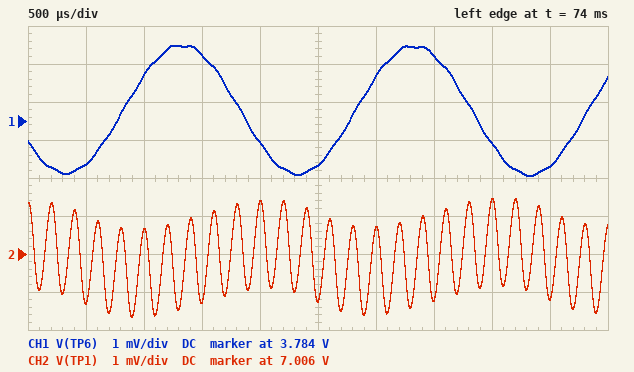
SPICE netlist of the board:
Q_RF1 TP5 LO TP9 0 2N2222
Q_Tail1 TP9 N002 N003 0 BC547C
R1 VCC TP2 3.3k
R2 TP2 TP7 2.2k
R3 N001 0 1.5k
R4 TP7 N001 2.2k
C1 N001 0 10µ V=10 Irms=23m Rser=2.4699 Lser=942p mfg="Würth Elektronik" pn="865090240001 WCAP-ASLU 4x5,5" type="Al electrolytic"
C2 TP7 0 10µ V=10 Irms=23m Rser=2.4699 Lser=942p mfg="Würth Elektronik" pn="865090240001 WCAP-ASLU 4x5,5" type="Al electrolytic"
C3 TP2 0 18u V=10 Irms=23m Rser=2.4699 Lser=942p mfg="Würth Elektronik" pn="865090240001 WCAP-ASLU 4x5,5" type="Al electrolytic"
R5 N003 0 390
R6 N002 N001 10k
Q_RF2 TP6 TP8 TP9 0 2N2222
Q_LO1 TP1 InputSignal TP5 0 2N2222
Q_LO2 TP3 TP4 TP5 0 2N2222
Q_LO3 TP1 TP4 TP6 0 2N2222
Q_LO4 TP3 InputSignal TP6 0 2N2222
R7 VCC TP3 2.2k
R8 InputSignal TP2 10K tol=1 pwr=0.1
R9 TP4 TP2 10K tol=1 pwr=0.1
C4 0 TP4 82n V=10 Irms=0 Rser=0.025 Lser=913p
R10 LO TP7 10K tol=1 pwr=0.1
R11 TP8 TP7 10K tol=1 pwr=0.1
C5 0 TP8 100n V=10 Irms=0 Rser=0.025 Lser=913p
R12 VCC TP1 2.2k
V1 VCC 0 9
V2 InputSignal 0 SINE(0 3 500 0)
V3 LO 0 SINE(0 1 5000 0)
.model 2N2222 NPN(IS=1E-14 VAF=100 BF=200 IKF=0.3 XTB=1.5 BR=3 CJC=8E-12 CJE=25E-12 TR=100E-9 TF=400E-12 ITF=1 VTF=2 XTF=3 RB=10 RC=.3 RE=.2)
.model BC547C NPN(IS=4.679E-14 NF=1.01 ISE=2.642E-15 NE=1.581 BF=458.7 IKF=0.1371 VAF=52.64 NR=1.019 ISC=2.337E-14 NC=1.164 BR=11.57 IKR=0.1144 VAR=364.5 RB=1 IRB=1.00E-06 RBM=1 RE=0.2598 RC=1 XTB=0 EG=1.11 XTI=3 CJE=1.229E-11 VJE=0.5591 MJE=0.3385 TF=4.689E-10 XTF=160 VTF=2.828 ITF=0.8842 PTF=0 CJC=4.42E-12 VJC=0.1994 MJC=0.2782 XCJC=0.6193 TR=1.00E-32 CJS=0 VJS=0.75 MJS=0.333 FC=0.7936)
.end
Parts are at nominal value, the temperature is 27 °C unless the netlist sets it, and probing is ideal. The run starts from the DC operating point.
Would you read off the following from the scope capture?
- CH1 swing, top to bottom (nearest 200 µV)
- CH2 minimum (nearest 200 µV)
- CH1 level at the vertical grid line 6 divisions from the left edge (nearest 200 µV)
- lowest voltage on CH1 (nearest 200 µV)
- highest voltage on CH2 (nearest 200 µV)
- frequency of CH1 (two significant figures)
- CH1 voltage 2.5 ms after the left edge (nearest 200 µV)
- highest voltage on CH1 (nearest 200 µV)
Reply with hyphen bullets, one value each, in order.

- 3.4 mV
- 7.0044 V
- 3.7852 V
- 3.7826 V
- 7.0074 V
- 500 Hz
- 3.7828 V
- 3.7860 V
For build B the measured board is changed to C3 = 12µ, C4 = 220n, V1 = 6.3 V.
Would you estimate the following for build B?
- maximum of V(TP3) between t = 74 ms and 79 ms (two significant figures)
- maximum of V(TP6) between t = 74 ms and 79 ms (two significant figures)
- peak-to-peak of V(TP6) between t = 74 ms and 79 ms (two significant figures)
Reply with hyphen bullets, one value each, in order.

- 6.3 V
- 2.5 V
- 2.2 mV
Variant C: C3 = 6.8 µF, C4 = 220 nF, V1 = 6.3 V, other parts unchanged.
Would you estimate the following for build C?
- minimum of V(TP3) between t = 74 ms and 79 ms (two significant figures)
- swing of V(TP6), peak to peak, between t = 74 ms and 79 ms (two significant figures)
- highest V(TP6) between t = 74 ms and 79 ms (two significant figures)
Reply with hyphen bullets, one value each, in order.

- 6.3 V
- 3.8 mV
- 2.5 V
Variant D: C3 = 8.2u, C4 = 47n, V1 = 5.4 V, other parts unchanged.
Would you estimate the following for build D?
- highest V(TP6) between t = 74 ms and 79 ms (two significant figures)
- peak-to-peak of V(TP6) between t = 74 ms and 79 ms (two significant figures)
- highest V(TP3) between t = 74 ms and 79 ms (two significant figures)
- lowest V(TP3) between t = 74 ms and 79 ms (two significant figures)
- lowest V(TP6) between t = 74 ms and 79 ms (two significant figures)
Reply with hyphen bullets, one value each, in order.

- 2.4 V
- 320 mV
- 5.4 V
- 5.2 V
- 2.1 V
